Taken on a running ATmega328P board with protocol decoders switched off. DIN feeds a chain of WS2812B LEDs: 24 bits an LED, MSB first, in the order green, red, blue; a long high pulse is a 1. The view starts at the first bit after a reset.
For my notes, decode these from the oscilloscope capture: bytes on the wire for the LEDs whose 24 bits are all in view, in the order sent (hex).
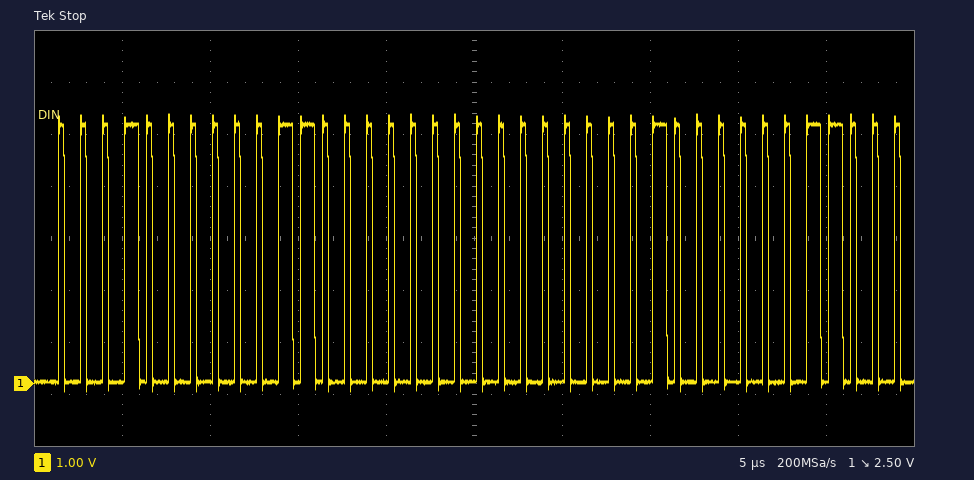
10 30 00
